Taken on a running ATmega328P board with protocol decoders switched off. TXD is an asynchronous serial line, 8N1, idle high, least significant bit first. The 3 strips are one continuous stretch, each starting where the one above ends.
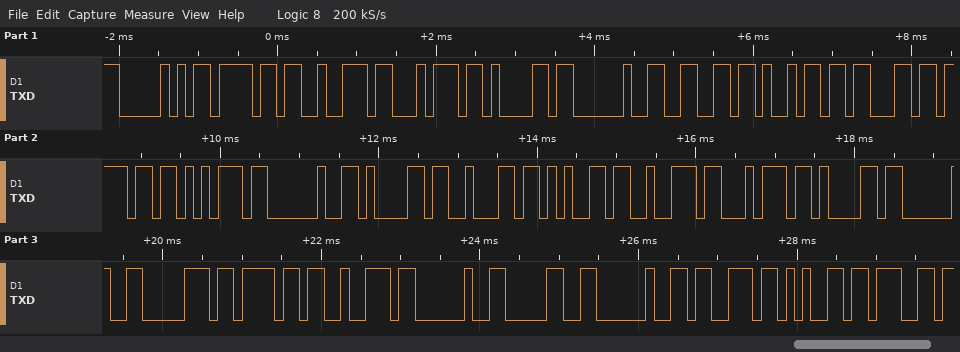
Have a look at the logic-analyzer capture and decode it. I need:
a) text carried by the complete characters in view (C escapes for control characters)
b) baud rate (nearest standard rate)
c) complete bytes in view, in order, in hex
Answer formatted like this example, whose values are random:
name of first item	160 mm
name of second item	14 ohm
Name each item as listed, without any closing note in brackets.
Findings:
text carried by the complete characters in view	"Porta ficou aberta por 0 seg"
baud rate	9600 baud
complete bytes in view, in order, in hex	50 6F 72 74 61 20 66 69 63 6F 75 20 61 62 65 72 74 61 20 70 6F 72 20 30 20 73 65 67
